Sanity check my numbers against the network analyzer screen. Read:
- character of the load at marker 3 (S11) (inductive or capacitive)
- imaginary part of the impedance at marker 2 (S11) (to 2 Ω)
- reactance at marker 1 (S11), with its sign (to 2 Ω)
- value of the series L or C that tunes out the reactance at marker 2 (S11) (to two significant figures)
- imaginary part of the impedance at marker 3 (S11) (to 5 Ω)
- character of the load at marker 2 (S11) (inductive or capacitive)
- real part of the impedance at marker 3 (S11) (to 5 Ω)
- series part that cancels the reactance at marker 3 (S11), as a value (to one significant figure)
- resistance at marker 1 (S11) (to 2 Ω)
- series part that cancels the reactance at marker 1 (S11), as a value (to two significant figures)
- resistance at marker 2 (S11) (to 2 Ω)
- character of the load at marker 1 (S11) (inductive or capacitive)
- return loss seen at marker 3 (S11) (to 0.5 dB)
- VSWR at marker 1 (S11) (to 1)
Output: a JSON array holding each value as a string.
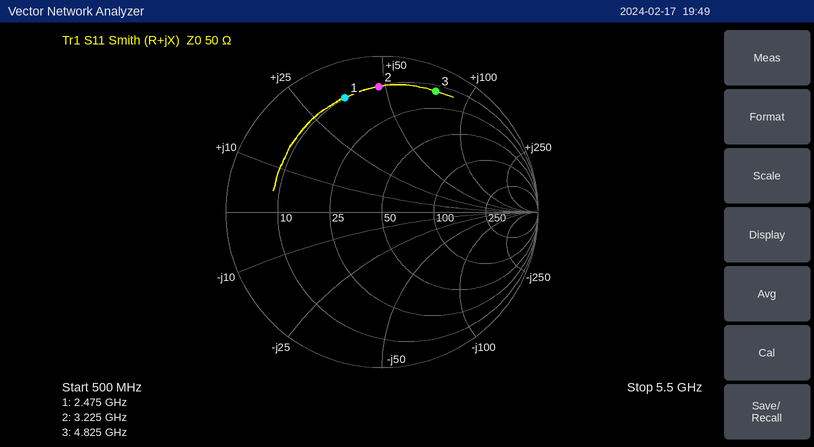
["inductive", "+48 Ω", "+36 Ω", "1.0 pF", "+75 Ω", "inductive", "15 Ω", "400 fF", "10 Ω", "1.8 pF", "10 Ω", "inductive", "1.5 dB", "8"]
